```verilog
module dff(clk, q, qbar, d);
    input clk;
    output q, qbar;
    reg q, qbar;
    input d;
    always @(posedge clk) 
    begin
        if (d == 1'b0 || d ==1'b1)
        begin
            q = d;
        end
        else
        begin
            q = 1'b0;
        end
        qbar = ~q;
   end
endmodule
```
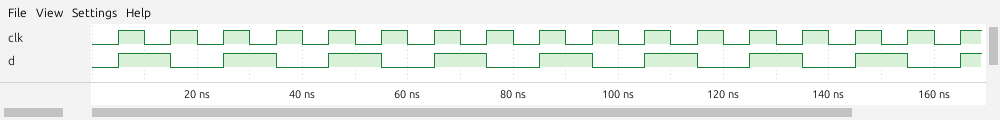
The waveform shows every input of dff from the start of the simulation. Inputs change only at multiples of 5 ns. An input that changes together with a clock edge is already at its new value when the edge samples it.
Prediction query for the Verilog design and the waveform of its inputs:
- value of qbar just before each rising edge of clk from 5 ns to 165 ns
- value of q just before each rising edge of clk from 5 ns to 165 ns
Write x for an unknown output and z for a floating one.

x 0 1 0 1 0 1 0 1 0 1 0 1 0 1 0 1
x 1 0 1 0 1 0 1 0 1 0 1 0 1 0 1 0
